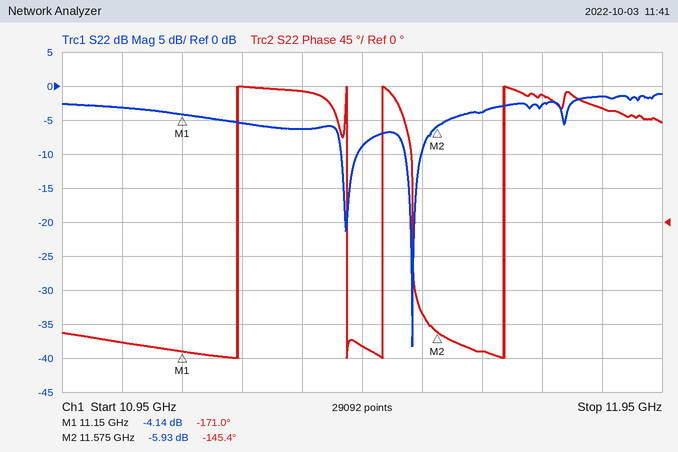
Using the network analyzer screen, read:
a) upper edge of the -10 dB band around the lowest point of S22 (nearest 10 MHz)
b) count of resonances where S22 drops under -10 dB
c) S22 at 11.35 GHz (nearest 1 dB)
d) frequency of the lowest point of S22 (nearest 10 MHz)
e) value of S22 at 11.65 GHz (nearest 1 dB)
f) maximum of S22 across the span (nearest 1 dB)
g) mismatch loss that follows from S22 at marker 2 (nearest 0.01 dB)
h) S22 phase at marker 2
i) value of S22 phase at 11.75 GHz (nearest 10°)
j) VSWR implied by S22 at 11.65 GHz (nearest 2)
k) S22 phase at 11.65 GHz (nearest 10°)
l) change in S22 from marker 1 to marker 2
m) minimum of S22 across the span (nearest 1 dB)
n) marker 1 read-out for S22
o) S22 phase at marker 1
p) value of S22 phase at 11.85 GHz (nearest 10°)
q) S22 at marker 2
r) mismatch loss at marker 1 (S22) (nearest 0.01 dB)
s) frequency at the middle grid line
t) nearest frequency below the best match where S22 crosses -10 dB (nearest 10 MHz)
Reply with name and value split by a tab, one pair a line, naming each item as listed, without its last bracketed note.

upper edge of the -10 dB band around the lowest point of S22	11.55 GHz
count of resonances where S22 drops under -10 dB	2
S22 at 11.35 GHz	-6 dB
frequency of the lowest point of S22	11.53 GHz
value of S22 at 11.65 GHz	-4 dB
maximum of S22 across the span	-1 dB
mismatch loss that follows from S22 at marker 2	1.28 dB
S22 phase at marker 2	-145.4°
value of S22 phase at 11.75 GHz	170°
VSWR implied by S22 at 11.65 GHz	4
S22 phase at 11.65 GHz	-170°
change in S22 from marker 1 to marker 2	-1.79 dB
minimum of S22 across the span	-38 dB
marker 1 read-out for S22	-4.14 dB
S22 phase at marker 1	-171.0°
value of S22 phase at 11.85 GHz	150°
S22 at marker 2	-5.93 dB
mismatch loss at marker 1 (S22)	2.11 dB
frequency at the middle grid line	11.45 GHz
nearest frequency below the best match where S22 crosses -10 dB	11.52 GHz
